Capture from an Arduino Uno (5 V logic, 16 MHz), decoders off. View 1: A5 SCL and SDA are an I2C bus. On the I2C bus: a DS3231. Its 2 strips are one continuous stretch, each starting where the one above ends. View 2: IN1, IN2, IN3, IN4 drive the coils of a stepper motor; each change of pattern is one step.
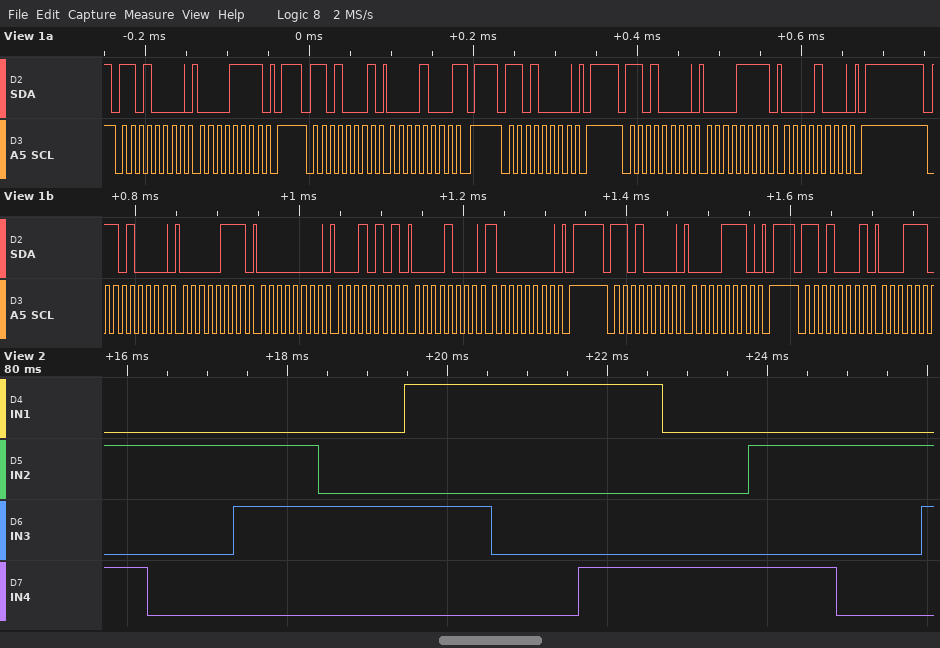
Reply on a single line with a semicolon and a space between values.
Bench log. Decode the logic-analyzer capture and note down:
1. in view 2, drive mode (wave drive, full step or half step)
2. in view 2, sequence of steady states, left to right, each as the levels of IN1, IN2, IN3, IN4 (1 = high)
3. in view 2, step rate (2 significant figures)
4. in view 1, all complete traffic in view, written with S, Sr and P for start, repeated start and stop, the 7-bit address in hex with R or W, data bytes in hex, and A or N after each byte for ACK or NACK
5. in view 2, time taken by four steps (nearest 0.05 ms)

half step; 0101 0100 0110 0010 1010 1000 1001 0001 0101 0100 0110; 930 steps/s; S 68W A 0F A P S 68R A 08 N P S 68W A P S 68W A 0F A 08 A P S 68W A 07 A 00 A 15 A 08 A 80 A P S 68W A 0E A P S 68R A; 4.30 ms
